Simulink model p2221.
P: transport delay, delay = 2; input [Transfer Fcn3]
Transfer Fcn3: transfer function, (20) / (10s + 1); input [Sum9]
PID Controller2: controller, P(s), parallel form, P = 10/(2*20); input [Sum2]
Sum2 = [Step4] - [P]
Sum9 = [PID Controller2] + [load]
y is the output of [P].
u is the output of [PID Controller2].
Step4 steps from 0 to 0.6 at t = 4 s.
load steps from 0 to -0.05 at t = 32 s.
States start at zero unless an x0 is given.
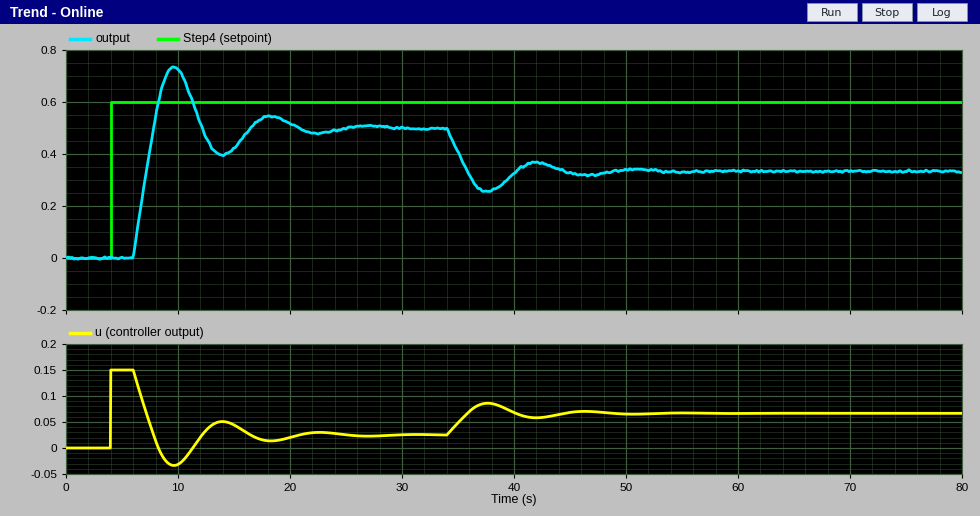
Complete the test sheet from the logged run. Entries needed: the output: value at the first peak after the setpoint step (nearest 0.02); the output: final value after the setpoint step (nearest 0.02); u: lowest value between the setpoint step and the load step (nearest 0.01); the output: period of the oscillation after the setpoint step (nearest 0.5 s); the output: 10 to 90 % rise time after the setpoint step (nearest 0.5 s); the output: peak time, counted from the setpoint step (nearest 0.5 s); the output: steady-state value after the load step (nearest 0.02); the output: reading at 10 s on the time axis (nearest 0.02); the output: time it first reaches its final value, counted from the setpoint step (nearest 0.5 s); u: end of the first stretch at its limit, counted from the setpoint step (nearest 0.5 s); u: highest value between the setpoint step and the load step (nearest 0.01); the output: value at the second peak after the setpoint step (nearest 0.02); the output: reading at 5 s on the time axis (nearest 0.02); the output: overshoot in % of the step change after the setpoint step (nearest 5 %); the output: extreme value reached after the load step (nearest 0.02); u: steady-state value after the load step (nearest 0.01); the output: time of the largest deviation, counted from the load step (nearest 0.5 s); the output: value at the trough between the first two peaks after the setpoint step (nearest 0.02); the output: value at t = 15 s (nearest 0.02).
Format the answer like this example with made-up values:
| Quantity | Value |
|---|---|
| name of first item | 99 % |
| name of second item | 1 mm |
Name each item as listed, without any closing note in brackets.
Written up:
| Quantity | Value |
|---|---|
| the output: value at the first peak after the setpoint step | 0.74 |
| the output: final value after the setpoint step | 0.50 |
| u: lowest value between the setpoint step and the load step | -0.03 |
| the output: period of the oscillation after the setpoint step | 8.5 s |
| the output: 10 to 90 % rise time after the setpoint step | 1.5 s |
| the output: peak time, counted from the setpoint step | 5.5 s |
| the output: steady-state value after the load step | 0.34 |
| the output: reading at 10 s on the time axis | 0.72 |
| the output: time it first reaches its final value, counted from the setpoint step | 4.0 s |
| u: end of the first stretch at its limit, counted from the setpoint step | 2.0 s |
| u: highest value between the setpoint step and the load step | 0.15 |
| the output: value at the second peak after the setpoint step | 0.54 |
| the output: reading at 5 s on the time axis | 0.00 |
| the output: overshoot in % of the step change after the setpoint step | 45 % |
| the output: extreme value reached after the load step | 0.26 |
| u: steady-state value after the load step | 0.07 |
| the output: time of the largest deviation, counted from the load step | 5.5 s |
| the output: value at the trough between the first two peaks after the setpoint step | 0.40 |
| the output: value at t = 15 s | 0.42 |
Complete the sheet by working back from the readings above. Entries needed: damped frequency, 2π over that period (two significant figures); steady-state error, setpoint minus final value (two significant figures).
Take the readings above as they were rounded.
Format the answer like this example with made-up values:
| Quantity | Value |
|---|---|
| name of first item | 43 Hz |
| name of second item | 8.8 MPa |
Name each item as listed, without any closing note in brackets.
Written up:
| Quantity | Value |
|---|---|
| damped frequency, 2π over that period | 0.74 rad/s |
| steady-state error, setpoint minus final value | 0.10 |
